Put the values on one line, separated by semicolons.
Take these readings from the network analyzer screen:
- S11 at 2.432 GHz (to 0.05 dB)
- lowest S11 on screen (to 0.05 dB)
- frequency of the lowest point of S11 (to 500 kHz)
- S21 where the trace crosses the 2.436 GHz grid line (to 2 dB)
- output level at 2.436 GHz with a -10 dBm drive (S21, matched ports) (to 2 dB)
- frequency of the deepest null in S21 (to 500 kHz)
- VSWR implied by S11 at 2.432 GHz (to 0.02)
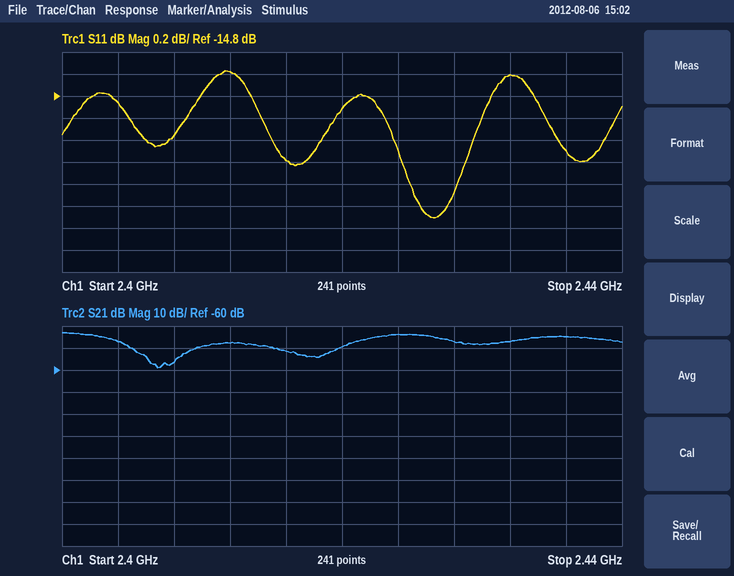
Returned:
-14.60 dB; -15.90 dB; 2.4265 GHz; -44 dB; -54 dBm; 2.4070 GHz; 1.46
